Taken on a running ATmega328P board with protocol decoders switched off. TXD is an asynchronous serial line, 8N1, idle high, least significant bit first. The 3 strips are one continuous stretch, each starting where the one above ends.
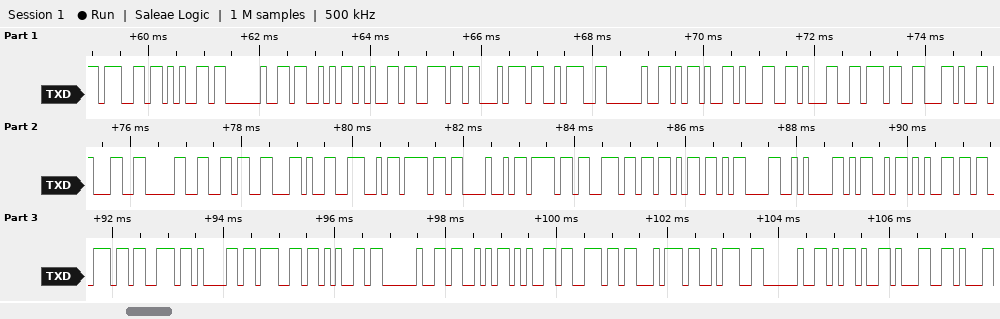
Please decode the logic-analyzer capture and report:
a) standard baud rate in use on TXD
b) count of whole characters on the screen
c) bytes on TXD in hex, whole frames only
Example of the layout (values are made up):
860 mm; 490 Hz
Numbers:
9600 baud; 42; 67 65 20 53 65 6E 74 3A 20 2D 31 31 37 2C 31 30 36 2C 4E 6F 48 6F 6E 6B 0D 0A 4D 65 73 73 61 67 65 20 53 65 6E 74 3A 20 2D 31
